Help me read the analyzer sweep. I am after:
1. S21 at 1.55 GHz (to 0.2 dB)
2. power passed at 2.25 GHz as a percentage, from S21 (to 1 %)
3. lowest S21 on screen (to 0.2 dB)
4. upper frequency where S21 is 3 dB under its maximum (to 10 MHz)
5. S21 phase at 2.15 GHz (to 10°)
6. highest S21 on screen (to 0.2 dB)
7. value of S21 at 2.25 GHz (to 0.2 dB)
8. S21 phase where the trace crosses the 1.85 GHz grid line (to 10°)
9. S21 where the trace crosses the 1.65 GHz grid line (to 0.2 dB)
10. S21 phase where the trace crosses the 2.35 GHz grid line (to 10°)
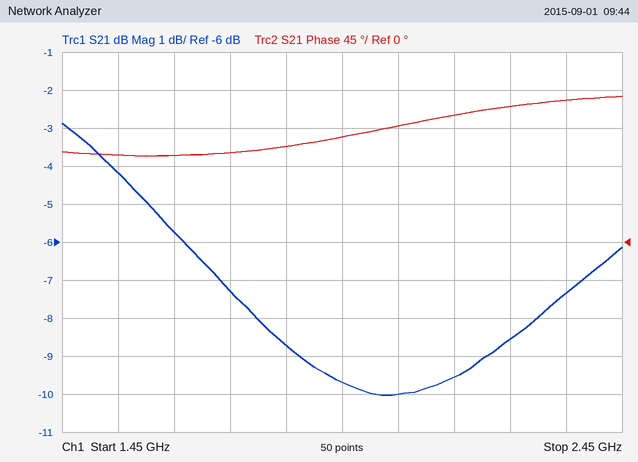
-4.2 dB
14 %
-10.0 dB
1.66 GHz
150°
-2.8 dB
-8.6 dB
110°
-5.8 dB
170°
